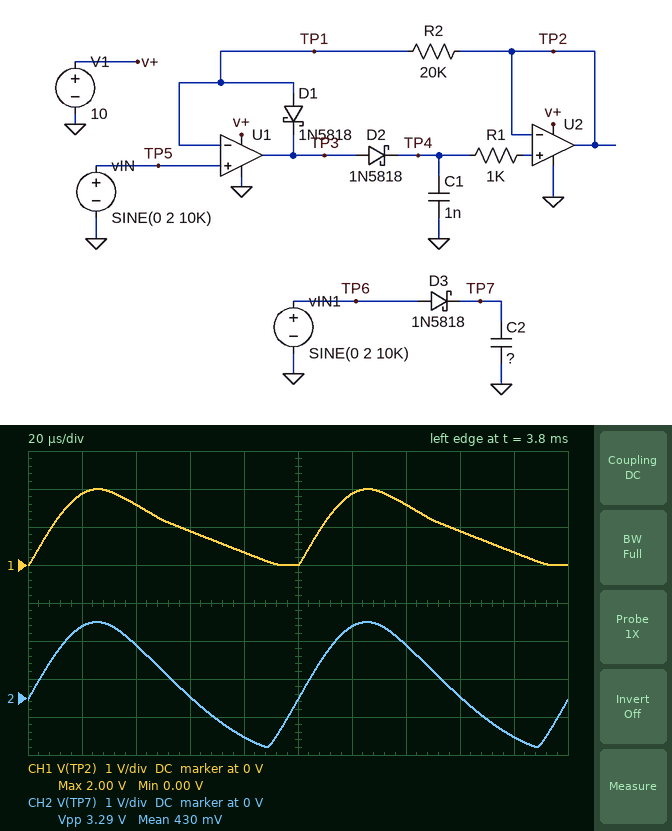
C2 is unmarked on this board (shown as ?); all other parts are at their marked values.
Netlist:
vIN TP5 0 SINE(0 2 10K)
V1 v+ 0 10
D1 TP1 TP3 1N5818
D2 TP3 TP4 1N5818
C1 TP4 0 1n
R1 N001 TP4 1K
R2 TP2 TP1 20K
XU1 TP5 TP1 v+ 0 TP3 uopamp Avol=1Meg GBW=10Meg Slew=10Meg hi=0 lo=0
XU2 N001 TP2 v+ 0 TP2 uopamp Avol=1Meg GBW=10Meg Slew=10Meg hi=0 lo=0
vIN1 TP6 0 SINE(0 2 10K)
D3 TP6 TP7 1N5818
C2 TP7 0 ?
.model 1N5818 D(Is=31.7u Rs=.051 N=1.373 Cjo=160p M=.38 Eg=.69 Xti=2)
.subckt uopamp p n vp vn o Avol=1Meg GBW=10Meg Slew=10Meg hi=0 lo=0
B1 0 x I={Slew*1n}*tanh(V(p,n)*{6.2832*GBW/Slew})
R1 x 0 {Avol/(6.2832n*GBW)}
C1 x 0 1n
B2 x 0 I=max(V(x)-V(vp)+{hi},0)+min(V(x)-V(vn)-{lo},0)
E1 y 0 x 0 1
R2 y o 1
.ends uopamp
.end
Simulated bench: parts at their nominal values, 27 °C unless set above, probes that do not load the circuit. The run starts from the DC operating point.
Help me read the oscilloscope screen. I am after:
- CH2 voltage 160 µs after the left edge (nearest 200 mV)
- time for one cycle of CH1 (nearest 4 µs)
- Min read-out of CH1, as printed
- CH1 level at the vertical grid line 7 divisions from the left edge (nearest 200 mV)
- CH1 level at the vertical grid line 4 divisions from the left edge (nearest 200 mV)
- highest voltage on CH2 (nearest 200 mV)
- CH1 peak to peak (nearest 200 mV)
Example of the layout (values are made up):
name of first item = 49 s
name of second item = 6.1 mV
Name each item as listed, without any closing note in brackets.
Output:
CH2 voltage 160 µs after the left edge = 0 V
time for one cycle of CH1 = 100 µs
Min read-out of CH1, as printed = 0.00 V
CH1 level at the vertical grid line 7 divisions from the left edge = 1.6 V
CH1 level at the vertical grid line 4 divisions from the left edge = 400 mV
highest voltage on CH2 = 2.0 V
CH1 peak to peak = 2.0 V
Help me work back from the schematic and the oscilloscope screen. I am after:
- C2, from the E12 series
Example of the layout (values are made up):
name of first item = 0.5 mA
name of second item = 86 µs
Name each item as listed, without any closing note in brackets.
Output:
C2, from the E12 series = 560 pF
